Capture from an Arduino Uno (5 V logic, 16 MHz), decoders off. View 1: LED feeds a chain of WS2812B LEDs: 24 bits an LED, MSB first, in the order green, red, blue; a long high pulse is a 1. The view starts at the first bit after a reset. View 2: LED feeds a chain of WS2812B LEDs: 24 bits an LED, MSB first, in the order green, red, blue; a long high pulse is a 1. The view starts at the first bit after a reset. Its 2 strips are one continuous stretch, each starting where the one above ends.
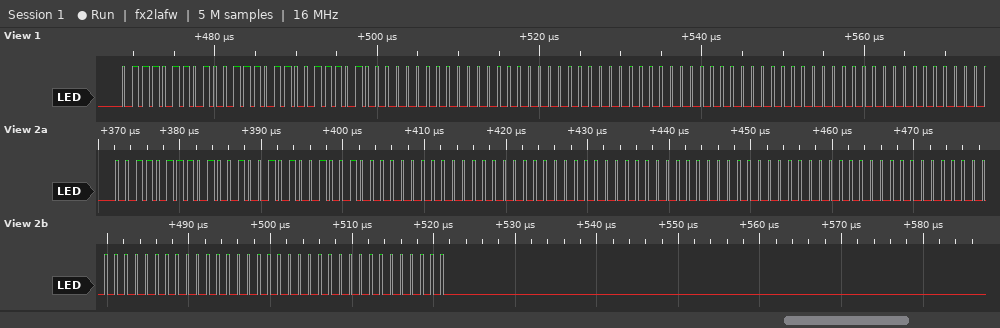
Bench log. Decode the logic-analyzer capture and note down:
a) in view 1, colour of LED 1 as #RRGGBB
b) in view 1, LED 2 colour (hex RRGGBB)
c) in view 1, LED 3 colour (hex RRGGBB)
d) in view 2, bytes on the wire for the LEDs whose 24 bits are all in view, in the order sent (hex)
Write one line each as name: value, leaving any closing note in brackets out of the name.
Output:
in view 1, colour of LED 1 as #RRGGBB: #9D769D
in view 1, LED 2 colour: #000000
in view 1, LED 3 colour: #000000
in view 2, bytes on the wire for the LEDs whose 24 bits are all in view, in the order sent: 37 49 49 00 00 00 00 00 00 00 00 00 00 00 00
